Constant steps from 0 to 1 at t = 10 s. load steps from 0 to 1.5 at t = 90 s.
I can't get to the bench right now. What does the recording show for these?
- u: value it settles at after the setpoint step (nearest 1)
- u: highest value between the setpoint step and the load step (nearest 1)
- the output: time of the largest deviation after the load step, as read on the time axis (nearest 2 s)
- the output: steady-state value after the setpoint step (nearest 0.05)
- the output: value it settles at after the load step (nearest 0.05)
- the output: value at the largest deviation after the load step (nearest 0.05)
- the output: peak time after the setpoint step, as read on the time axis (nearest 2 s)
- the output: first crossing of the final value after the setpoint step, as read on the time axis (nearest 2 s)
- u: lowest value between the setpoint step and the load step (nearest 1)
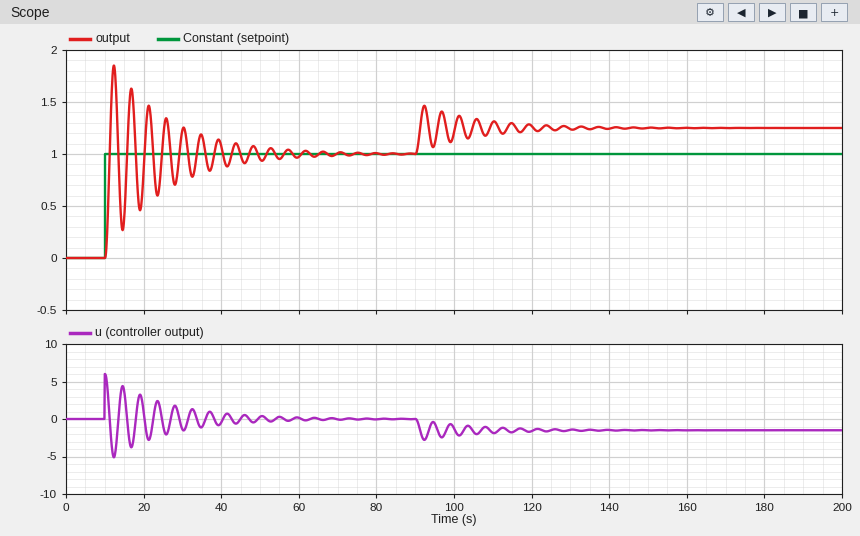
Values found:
0
6
92 s
1.00
1.25
1.45
12 s
12 s
-5
